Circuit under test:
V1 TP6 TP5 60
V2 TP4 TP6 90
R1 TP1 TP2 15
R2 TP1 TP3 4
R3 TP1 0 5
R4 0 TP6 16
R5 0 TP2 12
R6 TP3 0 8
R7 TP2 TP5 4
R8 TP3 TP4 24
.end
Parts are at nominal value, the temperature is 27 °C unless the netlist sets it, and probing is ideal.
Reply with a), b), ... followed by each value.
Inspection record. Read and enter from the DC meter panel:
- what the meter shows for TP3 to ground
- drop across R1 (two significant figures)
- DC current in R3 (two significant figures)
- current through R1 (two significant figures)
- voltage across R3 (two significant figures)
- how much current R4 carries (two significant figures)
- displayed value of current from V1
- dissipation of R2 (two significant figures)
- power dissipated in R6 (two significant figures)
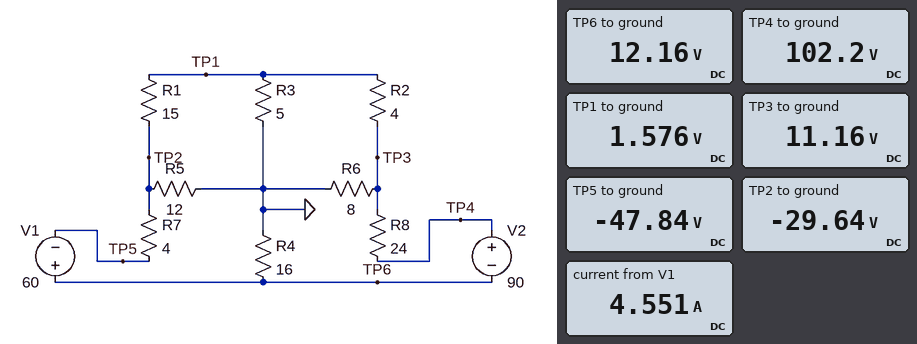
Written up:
a) 11.16 V
b) 31 V
c) 320 mA
d) 2.1 A
e) 1.6 V
f) 760 mA
g) 4.551 A
h) 23 W
i) 16 W
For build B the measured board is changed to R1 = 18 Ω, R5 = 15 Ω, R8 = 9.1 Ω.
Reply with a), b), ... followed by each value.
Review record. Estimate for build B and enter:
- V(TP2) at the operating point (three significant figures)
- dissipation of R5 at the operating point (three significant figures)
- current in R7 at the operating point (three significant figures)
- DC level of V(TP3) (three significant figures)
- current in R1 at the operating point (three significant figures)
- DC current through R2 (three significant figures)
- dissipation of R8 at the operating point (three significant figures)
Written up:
a) -46.0 V
b) 141 W
c) 5.92 A
d) 20.9 V
e) 2.85 A
f) 3.91 A
g) 387 W
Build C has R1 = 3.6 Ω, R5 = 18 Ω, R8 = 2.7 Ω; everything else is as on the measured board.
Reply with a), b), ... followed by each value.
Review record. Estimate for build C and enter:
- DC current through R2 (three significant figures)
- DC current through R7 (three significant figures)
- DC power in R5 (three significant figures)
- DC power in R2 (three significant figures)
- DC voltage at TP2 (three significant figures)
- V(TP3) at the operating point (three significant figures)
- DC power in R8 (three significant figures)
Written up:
a) 8.84 A
b) 11.5 A
c) 75.5 W
d) 313 W
e) -36.9 V
f) 32.4 V
g) 449 W
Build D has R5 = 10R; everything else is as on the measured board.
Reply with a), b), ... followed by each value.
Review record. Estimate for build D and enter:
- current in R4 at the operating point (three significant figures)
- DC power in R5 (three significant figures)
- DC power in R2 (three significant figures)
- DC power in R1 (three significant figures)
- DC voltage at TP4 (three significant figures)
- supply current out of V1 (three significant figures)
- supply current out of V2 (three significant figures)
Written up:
a) 863 mA
b) 75.0 W
c) 22.8 W
d) 57.9 W
e) 104 V
f) 4.70 A
g) 3.84 A
